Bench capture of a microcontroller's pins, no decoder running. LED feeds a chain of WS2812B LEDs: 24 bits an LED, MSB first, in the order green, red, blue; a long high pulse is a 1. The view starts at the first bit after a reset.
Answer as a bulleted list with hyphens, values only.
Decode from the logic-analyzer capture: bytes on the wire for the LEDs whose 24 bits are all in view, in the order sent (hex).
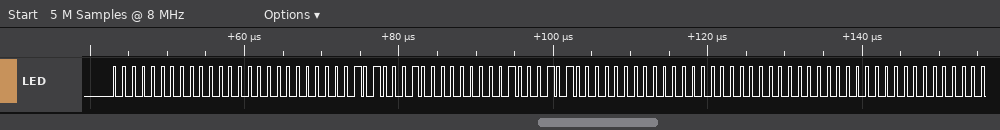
- 00 00 00 51 00 45 00 00 00
